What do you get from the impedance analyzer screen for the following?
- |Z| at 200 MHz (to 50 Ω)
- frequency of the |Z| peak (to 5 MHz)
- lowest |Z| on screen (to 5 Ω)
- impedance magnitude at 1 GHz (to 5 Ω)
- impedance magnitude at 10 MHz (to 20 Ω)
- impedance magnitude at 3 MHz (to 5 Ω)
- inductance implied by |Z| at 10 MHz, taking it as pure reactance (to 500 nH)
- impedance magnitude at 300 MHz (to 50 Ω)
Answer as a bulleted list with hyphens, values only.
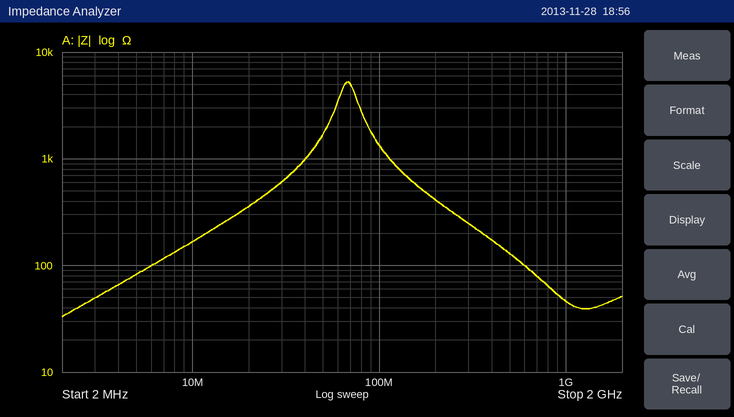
- 400 Ω
- 70 MHz
- 35 Ω
- 45 Ω
- 160 Ω
- 50 Ω
- 2.5 µH
- 250 Ω
